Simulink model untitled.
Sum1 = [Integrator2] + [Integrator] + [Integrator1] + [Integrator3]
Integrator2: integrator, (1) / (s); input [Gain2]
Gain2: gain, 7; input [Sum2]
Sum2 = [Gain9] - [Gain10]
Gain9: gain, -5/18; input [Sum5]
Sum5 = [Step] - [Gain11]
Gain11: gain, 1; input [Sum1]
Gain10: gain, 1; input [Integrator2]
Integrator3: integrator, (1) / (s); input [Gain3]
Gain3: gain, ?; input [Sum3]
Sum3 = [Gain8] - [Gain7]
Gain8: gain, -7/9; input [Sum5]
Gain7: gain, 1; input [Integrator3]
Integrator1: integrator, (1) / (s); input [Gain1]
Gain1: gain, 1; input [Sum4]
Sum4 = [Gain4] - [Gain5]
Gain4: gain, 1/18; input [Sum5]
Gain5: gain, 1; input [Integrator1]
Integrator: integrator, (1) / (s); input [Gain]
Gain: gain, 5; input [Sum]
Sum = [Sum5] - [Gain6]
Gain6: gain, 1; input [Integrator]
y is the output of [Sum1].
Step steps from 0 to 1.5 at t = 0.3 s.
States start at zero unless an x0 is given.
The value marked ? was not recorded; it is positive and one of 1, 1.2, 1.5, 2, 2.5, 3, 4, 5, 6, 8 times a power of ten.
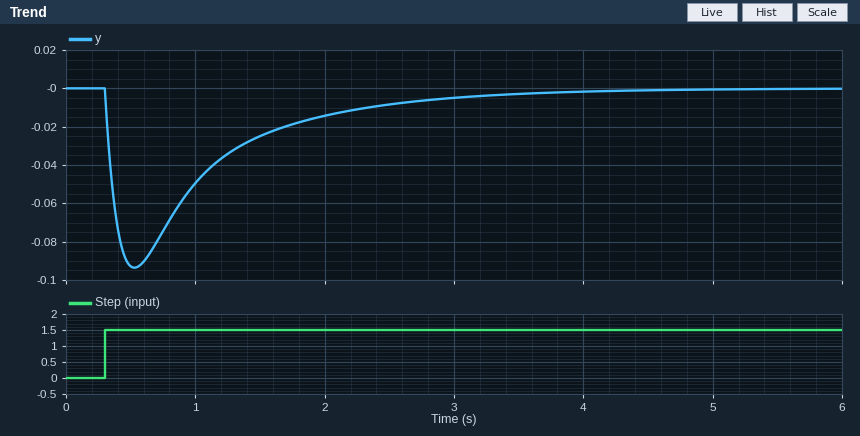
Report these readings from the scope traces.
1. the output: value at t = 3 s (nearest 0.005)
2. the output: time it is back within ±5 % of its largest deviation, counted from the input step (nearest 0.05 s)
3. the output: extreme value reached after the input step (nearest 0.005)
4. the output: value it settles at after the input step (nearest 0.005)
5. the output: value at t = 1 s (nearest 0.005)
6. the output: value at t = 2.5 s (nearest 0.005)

-0.005
2.75 s
-0.095
0.000
-0.050
-0.010
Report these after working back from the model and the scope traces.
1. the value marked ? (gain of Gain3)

5
